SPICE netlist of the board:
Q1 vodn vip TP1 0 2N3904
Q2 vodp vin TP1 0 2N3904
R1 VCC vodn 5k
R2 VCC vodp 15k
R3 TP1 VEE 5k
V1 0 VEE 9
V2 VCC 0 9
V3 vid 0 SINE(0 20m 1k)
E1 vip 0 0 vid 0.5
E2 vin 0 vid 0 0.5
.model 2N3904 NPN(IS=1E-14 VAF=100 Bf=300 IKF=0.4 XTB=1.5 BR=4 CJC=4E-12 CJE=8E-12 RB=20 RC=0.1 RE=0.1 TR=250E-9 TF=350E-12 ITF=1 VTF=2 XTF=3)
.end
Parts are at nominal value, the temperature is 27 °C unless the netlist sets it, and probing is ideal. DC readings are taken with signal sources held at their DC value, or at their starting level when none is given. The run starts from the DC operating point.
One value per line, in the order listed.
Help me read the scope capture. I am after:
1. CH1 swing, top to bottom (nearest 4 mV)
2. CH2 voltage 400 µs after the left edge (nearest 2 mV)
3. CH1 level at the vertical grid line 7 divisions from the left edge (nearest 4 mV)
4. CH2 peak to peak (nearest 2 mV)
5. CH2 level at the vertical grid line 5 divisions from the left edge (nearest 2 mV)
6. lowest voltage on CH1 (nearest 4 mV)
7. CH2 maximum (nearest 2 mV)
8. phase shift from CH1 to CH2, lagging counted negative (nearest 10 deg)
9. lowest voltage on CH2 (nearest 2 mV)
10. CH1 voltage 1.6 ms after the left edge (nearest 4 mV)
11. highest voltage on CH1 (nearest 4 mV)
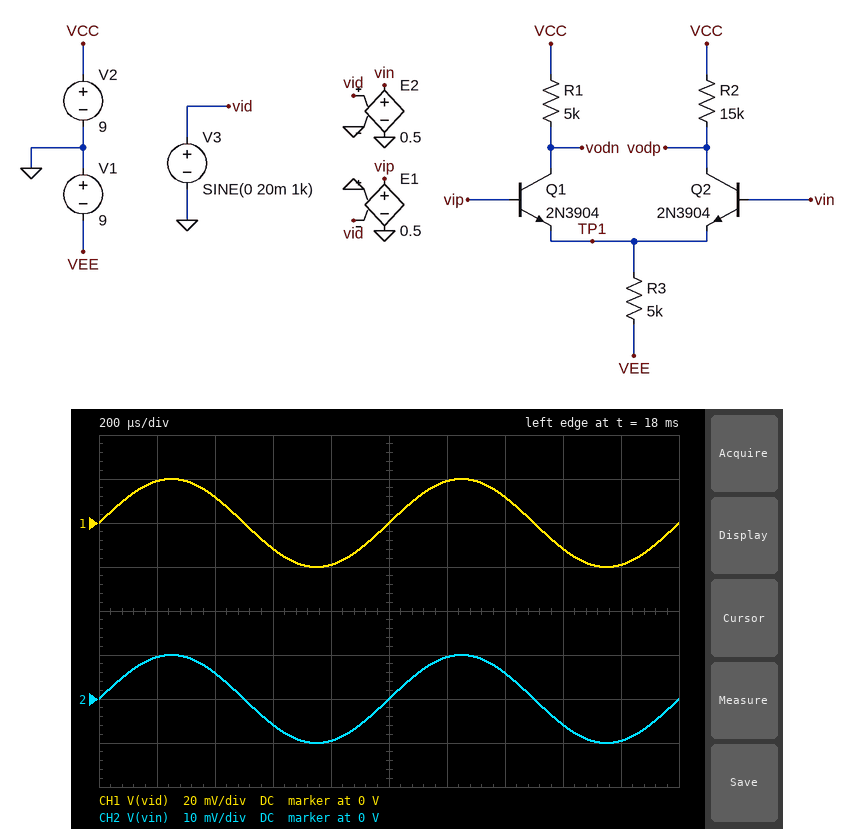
40 mV
6 mV
12 mV
20 mV
0 V
-20 mV
10 mV
0 deg
-10 mV
-12 mV
20 mV
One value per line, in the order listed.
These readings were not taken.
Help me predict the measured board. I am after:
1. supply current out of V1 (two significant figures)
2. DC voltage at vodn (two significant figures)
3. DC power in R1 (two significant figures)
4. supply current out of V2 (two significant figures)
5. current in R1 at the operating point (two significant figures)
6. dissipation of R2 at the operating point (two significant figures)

1.7 mA
4.1 V
4.7 mW
1.6 mA
970 µA
6.2 mW
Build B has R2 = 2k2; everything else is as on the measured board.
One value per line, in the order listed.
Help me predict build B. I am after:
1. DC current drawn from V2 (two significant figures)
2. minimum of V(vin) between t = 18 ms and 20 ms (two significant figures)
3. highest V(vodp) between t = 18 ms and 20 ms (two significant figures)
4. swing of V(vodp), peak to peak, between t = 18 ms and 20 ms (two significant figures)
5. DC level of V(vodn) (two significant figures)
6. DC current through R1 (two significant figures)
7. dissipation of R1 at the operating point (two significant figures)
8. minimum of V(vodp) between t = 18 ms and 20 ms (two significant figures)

1.7 mA
-10 mV
7.8 V
1.3 V
4.9 V
820 µA
3.4 mW
6.5 V
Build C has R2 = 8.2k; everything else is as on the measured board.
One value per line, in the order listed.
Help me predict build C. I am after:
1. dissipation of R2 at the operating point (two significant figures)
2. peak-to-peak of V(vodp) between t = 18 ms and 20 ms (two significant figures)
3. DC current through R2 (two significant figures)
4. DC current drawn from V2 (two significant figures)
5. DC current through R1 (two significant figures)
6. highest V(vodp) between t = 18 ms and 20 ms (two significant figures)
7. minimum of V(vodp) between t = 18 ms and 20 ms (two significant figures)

5.5 mW
4.8 V
820 µA
1.7 mA
840 µA
4.6 V
-140 mV
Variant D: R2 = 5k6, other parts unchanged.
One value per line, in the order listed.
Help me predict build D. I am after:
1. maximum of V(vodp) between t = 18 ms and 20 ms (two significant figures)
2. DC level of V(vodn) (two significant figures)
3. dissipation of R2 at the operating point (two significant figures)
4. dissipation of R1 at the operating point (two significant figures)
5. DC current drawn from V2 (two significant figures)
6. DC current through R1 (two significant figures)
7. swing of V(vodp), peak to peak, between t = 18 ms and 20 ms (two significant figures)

6.0 V
4.8 V
3.9 mW
3.5 mW
1.7 mA
830 µA
3.3 V
